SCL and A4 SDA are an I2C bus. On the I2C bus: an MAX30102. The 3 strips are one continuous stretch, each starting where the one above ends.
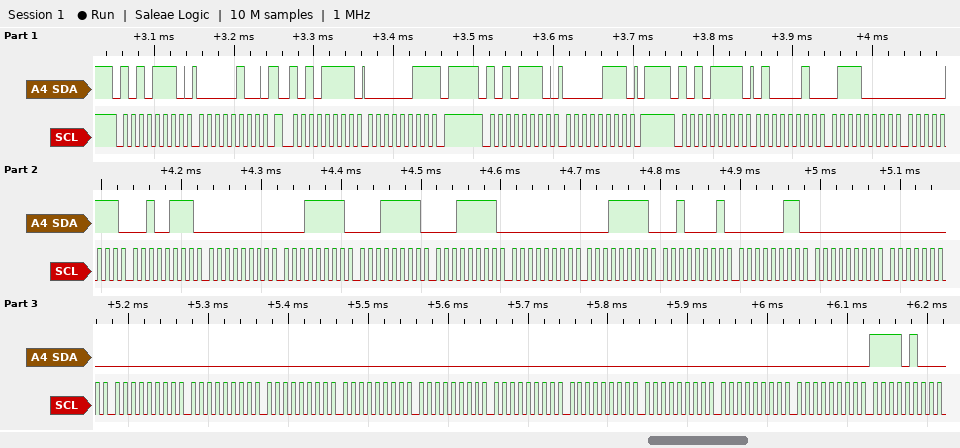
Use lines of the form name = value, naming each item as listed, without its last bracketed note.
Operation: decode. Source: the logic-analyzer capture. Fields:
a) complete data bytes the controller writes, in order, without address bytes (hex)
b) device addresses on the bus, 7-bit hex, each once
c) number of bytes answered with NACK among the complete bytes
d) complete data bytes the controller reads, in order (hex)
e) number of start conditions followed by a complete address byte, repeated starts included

complete data bytes the controller writes, in order, without address bytes = 04 07
device addresses on the bus, 7-bit hex, each once = 0x57
number of bytes answered with NACK among the complete bytes = 1
complete data bytes the controller reads, in order = 03 42 70 07 27 00 1F 1F 1F 00 1F 21 03 00 00 00 00 00 00 00 00 00 00 00 00 F4
number of start conditions followed by a complete address byte, repeated starts included = 4
